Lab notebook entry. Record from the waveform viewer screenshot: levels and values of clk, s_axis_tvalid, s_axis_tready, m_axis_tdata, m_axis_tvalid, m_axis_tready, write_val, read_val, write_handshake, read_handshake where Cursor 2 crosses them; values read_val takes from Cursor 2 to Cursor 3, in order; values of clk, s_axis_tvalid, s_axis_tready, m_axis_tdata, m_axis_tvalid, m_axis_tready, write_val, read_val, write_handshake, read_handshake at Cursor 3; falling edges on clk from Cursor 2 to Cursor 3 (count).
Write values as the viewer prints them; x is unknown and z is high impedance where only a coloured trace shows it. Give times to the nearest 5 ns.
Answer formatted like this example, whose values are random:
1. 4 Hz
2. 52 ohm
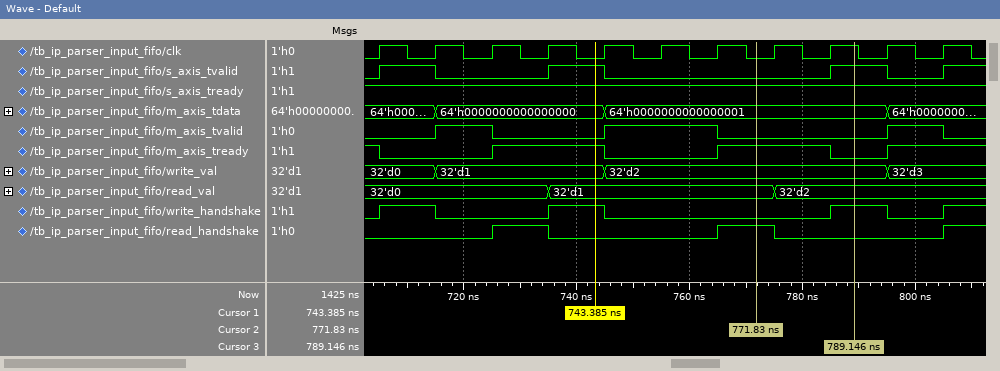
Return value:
1. clk=0, s_axis_tvalid=0, s_axis_tready=1, m_axis_tdata=64'h0000000000000001, m_axis_tvalid=0, m_axis_tready=1, write_val=32'd2, read_val=32'd1, write_handshake=0, read_handshake=1
2. 32'd1, 32'd2
3. clk=1, s_axis_tvalid=1, s_axis_tready=1, m_axis_tdata=64'h0000000000000001, m_axis_tvalid=0, m_axis_tready=0, write_val=32'd2, read_val=32'd2, write_handshake=1, read_handshake=0
4. 1
